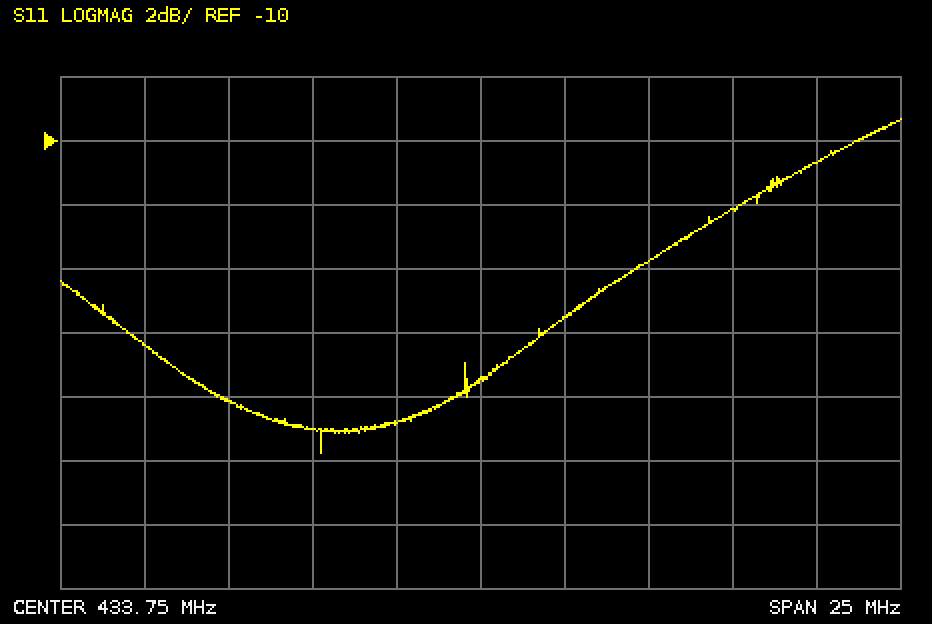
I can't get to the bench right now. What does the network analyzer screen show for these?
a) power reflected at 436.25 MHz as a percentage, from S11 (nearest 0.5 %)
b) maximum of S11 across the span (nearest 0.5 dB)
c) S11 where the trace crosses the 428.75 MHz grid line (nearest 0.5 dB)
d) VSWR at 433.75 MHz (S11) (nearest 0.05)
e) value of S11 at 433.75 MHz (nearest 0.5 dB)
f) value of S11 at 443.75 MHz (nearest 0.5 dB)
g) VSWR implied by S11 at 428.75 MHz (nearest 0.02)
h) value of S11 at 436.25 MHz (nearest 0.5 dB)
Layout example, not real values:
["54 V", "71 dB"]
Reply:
["3.0 %", "-9.5 dB", "-19.0 dB", "1.30", "-17.5 dB", "-10.5 dB", "1.26", "-15.5 dB"]
